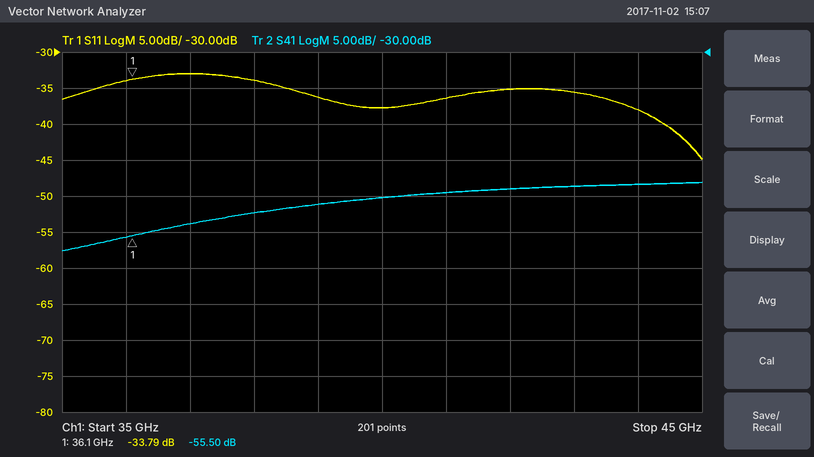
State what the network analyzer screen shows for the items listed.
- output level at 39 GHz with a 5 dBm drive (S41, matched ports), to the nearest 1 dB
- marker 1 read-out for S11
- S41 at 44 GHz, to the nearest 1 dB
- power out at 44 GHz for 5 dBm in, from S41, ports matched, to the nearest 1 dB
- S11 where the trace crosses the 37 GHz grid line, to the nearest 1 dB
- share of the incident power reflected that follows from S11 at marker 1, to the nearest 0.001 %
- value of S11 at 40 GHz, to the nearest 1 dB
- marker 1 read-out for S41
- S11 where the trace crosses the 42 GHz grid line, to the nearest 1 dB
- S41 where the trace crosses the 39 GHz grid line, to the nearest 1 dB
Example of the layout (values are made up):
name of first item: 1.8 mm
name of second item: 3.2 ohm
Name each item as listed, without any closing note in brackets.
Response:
output level at 39 GHz with a 5 dBm drive (S41, matched ports), to the nearest 1 dB: -46 dBm
marker 1 read-out for S11: -33.79 dB
S41 at 44 GHz, to the nearest 1 dB: -48 dB
power out at 44 GHz for 5 dBm in, from S41, ports matched, to the nearest 1 dB: -43 dBm
S11 where the trace crosses the 37 GHz grid line, to the nearest 1 dB: -33 dB
share of the incident power reflected that follows from S11 at marker 1, to the nearest 0.001 %: 0.042 %
value of S11 at 40 GHz, to the nearest 1 dB: -38 dB
marker 1 read-out for S41: -55.50 dB
S11 where the trace crosses the 42 GHz grid line, to the nearest 1 dB: -35 dB
S41 where the trace crosses the 39 GHz grid line, to the nearest 1 dB: -51 dB
